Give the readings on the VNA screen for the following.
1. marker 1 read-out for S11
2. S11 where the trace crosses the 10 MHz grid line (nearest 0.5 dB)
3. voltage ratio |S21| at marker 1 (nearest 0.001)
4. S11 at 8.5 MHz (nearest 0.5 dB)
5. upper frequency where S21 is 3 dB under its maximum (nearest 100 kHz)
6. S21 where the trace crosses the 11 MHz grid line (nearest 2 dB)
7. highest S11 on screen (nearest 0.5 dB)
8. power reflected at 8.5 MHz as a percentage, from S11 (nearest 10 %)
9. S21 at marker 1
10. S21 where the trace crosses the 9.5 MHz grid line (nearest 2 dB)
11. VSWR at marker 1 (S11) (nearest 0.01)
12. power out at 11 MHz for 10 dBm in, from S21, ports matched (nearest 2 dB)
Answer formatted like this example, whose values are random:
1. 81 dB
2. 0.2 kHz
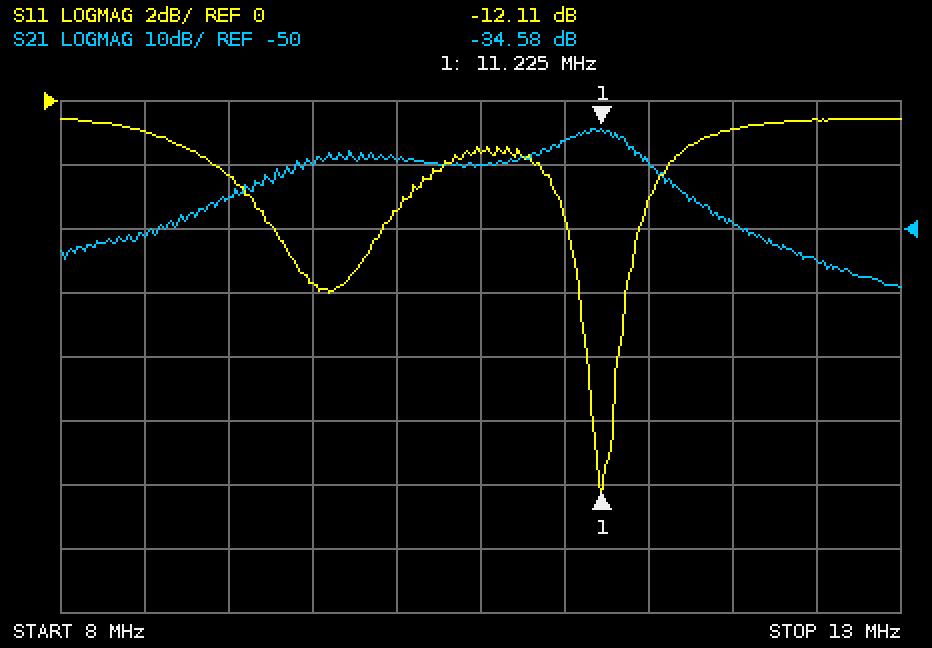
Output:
1. -12.11 dB
2. -3.5 dB
3. 0.019
4. -1.0 dB
5. 11.4 MHz
6. -36 dB
7. -0.5 dB
8. 80 %
9. -34.58 dB
10. -40 dB
11. 1.66
12. -26 dBm
